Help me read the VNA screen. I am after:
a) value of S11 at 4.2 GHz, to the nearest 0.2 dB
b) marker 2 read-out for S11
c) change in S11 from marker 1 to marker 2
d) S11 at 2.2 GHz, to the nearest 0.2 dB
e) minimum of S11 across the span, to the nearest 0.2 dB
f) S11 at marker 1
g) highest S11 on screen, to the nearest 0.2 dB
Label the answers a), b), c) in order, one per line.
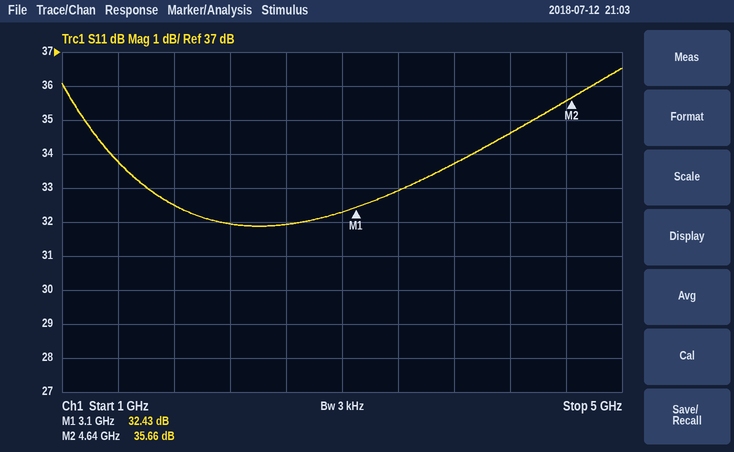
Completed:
a) 34.6 dB
b) 35.66 dB
c) 3.23 dB
d) 32.0 dB
e) 31.8 dB
f) 32.43 dB
g) 36.6 dB
